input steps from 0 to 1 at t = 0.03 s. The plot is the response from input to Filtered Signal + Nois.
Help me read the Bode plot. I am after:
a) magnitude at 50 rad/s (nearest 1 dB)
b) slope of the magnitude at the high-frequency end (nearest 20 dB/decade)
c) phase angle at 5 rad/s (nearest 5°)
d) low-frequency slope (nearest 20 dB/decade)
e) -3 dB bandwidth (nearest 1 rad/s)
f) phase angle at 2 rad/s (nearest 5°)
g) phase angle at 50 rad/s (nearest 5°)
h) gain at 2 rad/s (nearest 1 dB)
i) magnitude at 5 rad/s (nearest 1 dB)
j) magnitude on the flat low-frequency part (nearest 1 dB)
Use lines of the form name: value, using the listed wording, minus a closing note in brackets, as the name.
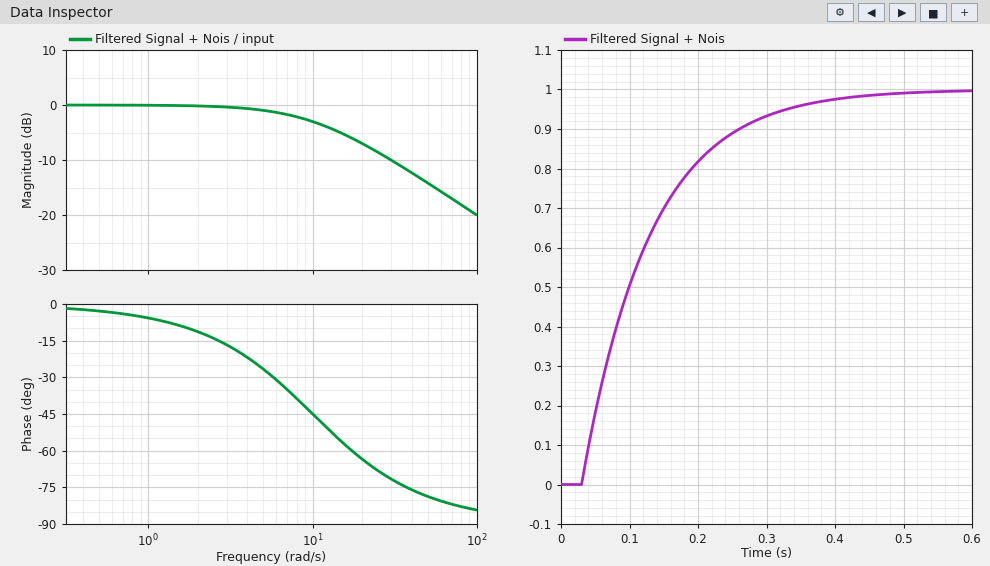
magnitude at 50 rad/s: -14 dB
slope of the magnitude at the high-frequency end: -20 dB/decade
phase angle at 5 rad/s: -25°
low-frequency slope: 0 dB/decade
-3 dB bandwidth: 10 rad/s
phase angle at 2 rad/s: -10°
phase angle at 50 rad/s: -80°
gain at 2 rad/s: 0 dB
magnitude at 5 rad/s: -1 dB
magnitude on the flat low-frequency part: 0 dB
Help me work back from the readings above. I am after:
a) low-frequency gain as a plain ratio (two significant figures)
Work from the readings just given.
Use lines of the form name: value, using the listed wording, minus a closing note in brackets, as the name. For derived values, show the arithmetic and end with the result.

low-frequency gain as a plain ratio: 10^(0 / 20) = 1.0
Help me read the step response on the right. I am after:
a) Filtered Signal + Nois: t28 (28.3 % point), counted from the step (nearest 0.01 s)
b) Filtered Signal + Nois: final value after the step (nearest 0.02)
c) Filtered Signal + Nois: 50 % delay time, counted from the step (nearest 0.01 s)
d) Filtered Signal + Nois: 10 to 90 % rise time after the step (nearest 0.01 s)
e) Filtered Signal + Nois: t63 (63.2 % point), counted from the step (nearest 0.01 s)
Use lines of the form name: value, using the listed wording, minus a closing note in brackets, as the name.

Filtered Signal + Nois: t28 (28.3 % point), counted from the step: 0.03 s
Filtered Signal + Nois: final value after the step: 1.00
Filtered Signal + Nois: 50 % delay time, counted from the step: 0.07 s
Filtered Signal + Nois: 10 to 90 % rise time after the step: 0.22 s
Filtered Signal + Nois: t63 (63.2 % point), counted from the step: 0.10 s
